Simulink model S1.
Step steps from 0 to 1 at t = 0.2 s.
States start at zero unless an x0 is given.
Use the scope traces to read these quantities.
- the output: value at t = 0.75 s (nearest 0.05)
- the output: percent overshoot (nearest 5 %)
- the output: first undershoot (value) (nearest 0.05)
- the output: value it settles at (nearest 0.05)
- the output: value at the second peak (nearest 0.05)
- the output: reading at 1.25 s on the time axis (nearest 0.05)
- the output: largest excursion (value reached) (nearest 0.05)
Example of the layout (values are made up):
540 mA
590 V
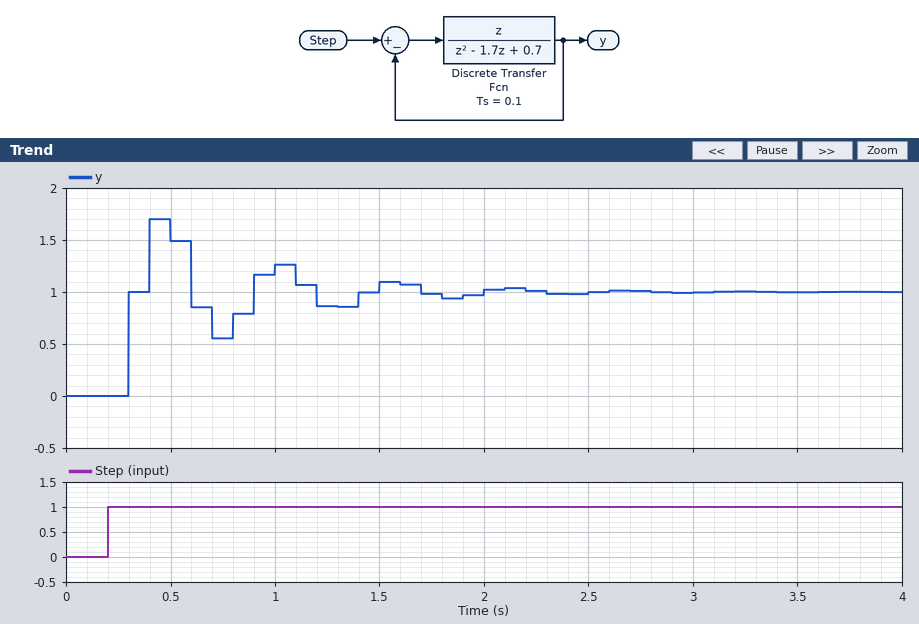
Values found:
0.55
70 %
0.55
1.00
1.25
0.85
1.70
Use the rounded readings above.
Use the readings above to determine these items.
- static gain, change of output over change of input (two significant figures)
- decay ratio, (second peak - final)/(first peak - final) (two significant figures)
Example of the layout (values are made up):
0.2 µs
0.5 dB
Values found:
1.0
0.36
